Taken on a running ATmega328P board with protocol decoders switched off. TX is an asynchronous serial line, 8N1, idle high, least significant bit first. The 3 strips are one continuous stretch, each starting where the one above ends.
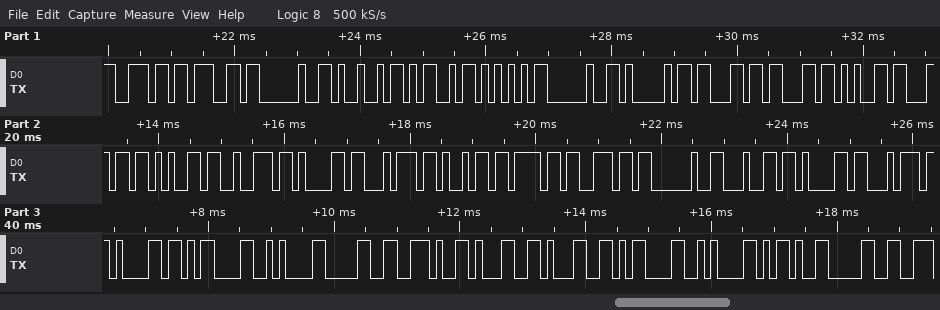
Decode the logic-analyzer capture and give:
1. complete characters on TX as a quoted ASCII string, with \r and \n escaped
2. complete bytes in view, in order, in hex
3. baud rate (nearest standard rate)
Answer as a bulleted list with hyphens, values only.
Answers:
- "ng IMU Acceleration data\r\n0.11\r\n-0"
- 6E 67 20 49 4D 55 20 41 63 63 65 6C 65 72 61 74 69 6F 6E 20 64 61 74 61 0D 0A 30 2E 31 31 0D 0A 2D 30
- 9600 baud
